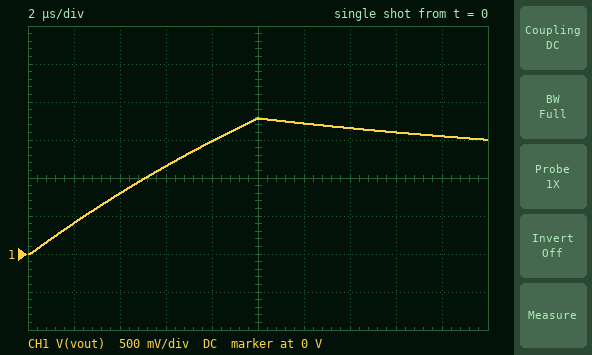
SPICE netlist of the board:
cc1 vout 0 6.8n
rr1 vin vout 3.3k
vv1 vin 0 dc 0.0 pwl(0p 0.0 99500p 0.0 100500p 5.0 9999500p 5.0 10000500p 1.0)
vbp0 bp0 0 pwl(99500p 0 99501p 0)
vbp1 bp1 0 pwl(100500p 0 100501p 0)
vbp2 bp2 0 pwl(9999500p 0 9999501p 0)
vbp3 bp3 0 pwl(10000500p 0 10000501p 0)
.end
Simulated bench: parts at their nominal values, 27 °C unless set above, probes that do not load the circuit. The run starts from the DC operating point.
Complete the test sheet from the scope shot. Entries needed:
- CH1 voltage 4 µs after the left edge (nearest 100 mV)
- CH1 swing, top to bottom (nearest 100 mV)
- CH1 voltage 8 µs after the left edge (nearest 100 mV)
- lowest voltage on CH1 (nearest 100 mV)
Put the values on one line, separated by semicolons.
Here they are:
800 mV; 1.8 V; 1.5 V; 0 V
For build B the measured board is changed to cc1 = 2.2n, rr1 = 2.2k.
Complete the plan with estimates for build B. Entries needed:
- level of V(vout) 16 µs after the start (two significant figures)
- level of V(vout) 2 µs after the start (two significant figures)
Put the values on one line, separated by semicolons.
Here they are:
2.0 V; 1.6 V
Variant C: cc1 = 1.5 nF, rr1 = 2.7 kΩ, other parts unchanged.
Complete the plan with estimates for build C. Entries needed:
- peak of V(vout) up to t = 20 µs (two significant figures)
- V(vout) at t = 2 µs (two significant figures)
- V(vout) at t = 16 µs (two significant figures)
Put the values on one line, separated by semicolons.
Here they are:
4.6 V; 1.9 V; 1.8 V
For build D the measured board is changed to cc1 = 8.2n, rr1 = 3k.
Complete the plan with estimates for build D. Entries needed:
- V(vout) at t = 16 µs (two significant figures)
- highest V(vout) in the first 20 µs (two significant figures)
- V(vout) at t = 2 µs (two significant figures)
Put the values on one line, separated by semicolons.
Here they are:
1.5 V; 1.7 V; 370 mV
